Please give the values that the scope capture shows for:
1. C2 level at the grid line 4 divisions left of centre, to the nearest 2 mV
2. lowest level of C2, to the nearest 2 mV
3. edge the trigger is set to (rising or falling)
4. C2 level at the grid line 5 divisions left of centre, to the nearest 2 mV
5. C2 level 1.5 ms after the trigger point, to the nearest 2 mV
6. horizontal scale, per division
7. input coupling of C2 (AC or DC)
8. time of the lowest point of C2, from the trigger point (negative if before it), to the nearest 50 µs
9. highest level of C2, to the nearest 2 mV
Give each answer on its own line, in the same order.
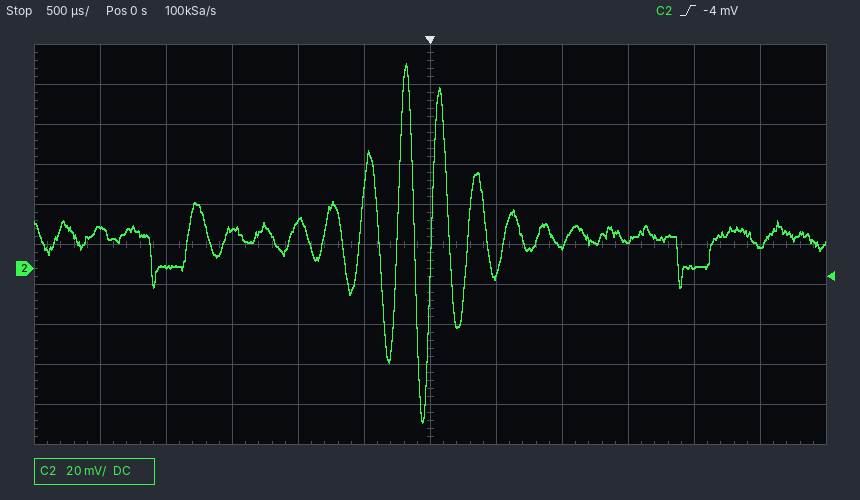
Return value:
0 mV
-76 mV
rising
20 mV
14 mV
500 µs
DC
-50 µs
102 mV
